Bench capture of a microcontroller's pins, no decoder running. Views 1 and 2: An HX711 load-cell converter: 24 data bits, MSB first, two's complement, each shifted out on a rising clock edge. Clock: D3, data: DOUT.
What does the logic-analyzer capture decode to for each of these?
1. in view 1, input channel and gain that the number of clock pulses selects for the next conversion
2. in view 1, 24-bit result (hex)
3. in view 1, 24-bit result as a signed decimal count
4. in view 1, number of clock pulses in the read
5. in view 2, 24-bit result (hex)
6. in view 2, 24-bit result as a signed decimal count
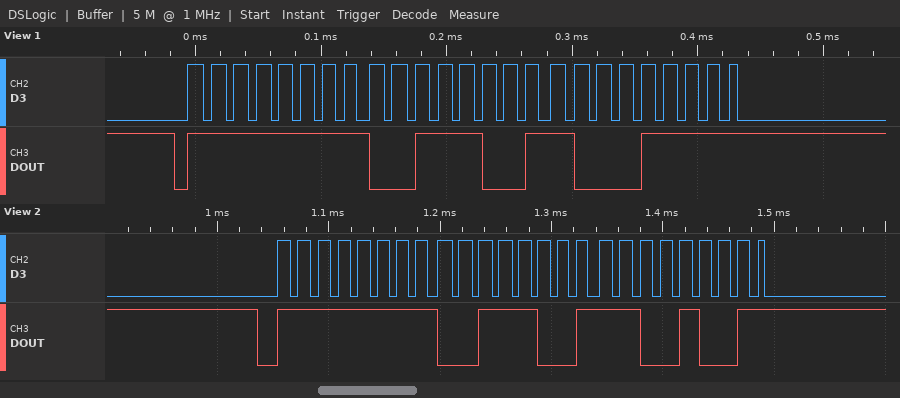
channel A, gain 128
0xFF398F
-50801
25
0xFF39C9
-50743
